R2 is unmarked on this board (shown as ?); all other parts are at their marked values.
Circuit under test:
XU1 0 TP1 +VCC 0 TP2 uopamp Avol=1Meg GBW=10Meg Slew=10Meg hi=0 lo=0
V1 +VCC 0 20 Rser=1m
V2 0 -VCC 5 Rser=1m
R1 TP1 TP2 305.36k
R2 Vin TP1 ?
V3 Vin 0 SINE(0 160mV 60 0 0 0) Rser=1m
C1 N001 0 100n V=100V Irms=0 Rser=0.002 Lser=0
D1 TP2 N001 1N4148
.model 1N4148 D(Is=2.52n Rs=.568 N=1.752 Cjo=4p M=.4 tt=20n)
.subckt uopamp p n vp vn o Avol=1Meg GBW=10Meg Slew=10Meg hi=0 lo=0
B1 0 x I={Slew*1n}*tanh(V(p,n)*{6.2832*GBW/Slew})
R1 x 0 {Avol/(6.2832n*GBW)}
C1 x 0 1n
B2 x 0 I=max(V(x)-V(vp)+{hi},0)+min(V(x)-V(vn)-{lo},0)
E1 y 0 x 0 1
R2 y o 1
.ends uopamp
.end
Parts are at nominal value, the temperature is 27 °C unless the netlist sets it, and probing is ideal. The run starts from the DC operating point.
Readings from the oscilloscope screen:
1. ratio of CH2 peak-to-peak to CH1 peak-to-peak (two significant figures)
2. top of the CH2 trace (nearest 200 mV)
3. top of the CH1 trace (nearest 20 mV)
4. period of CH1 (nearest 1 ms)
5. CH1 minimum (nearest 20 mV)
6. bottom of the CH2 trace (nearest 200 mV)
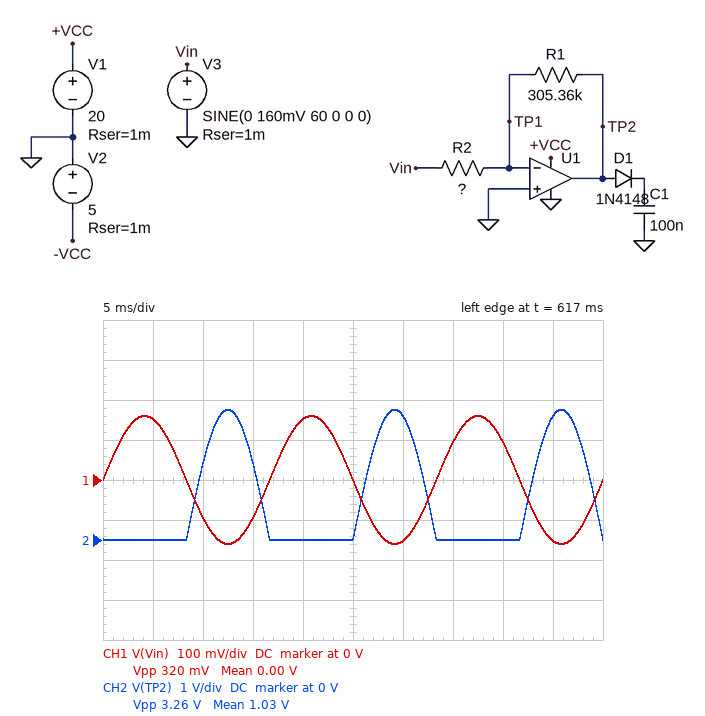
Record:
10
3.2 V
160 mV
17 ms
-160 mV
0 V
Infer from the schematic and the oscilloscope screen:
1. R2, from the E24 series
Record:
15 kΩ
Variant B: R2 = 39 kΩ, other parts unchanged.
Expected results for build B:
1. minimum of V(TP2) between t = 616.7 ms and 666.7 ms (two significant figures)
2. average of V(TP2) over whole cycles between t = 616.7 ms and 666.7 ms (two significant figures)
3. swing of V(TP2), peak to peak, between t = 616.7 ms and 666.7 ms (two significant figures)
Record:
-7.1 mV
400 mV
1.3 V
